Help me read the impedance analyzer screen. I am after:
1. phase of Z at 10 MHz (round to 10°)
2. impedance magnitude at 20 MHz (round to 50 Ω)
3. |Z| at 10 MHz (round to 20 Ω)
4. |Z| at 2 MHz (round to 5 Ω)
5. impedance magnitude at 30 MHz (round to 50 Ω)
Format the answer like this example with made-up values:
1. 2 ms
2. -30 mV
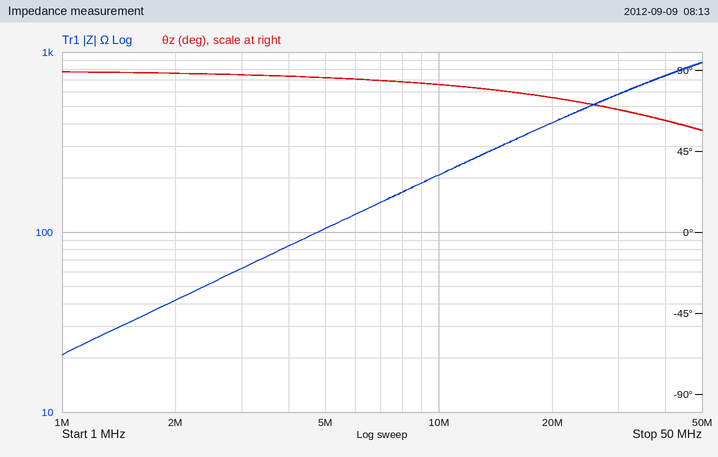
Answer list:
1. 80°
2. 400 Ω
3. 200 Ω
4. 40 Ω
5. 600 Ω
